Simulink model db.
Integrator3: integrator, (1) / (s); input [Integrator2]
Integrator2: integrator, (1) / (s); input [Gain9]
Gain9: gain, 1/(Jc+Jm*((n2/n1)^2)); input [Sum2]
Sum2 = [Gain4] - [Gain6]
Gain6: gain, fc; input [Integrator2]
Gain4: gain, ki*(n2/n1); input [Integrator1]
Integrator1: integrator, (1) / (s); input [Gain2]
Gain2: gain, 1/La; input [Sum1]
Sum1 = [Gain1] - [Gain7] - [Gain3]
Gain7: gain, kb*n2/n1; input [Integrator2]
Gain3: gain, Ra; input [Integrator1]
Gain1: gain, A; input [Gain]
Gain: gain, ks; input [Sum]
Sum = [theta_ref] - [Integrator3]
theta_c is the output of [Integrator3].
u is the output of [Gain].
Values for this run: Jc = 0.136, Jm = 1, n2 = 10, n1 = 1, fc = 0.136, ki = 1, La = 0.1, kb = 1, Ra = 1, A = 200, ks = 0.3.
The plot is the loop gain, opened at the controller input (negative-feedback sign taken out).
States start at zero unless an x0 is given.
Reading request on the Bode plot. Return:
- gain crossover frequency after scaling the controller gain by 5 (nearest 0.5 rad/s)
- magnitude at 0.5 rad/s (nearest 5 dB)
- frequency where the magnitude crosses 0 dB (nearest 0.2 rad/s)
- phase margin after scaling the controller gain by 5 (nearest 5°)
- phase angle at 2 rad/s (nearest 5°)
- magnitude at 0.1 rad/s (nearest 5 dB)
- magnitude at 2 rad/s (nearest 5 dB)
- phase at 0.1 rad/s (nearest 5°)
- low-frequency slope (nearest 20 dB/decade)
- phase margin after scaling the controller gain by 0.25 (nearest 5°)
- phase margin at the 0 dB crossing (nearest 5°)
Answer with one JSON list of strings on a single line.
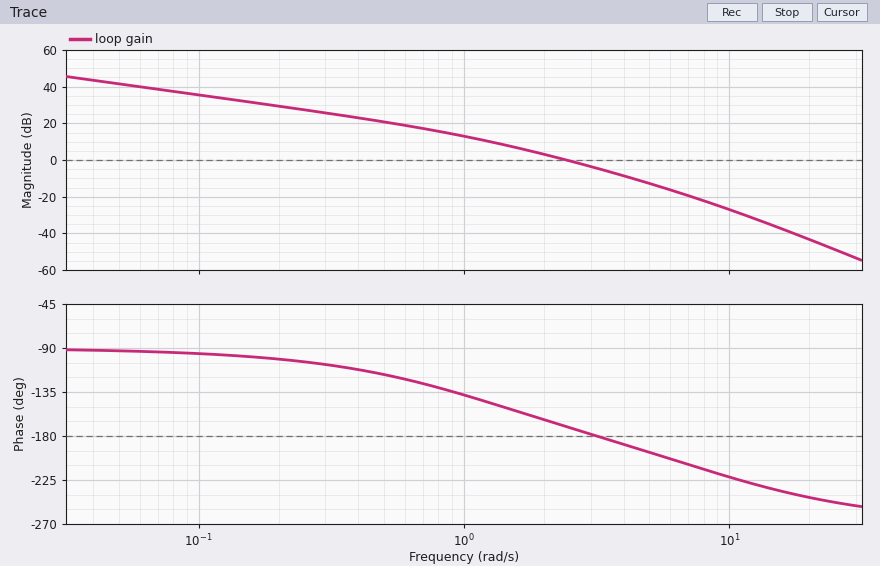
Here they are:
["5.5 rad/s", "20 dB", "2.4 rad/s", "-20°", "-165°", "35 dB", "5 dB", "-95°", "-20 dB/decade", "40°", "10°"]
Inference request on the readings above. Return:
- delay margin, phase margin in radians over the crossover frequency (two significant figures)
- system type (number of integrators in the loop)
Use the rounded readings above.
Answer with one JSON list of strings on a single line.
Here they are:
["0.073 s", "1"]
